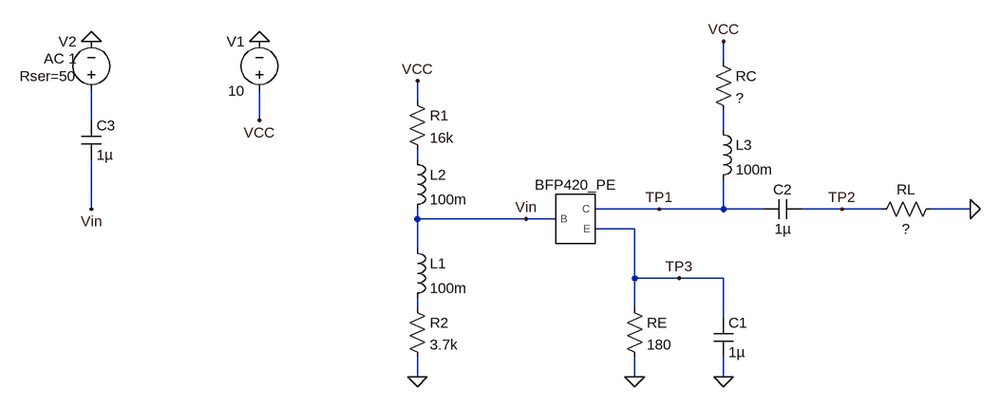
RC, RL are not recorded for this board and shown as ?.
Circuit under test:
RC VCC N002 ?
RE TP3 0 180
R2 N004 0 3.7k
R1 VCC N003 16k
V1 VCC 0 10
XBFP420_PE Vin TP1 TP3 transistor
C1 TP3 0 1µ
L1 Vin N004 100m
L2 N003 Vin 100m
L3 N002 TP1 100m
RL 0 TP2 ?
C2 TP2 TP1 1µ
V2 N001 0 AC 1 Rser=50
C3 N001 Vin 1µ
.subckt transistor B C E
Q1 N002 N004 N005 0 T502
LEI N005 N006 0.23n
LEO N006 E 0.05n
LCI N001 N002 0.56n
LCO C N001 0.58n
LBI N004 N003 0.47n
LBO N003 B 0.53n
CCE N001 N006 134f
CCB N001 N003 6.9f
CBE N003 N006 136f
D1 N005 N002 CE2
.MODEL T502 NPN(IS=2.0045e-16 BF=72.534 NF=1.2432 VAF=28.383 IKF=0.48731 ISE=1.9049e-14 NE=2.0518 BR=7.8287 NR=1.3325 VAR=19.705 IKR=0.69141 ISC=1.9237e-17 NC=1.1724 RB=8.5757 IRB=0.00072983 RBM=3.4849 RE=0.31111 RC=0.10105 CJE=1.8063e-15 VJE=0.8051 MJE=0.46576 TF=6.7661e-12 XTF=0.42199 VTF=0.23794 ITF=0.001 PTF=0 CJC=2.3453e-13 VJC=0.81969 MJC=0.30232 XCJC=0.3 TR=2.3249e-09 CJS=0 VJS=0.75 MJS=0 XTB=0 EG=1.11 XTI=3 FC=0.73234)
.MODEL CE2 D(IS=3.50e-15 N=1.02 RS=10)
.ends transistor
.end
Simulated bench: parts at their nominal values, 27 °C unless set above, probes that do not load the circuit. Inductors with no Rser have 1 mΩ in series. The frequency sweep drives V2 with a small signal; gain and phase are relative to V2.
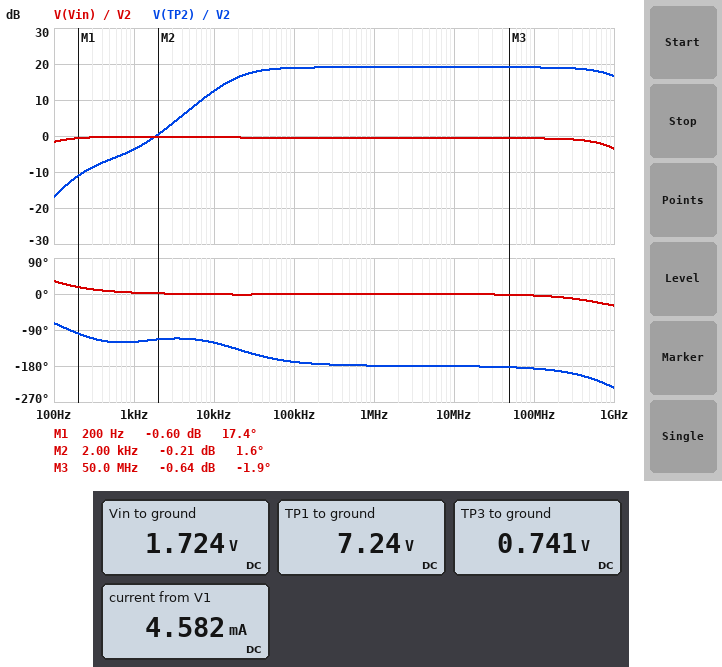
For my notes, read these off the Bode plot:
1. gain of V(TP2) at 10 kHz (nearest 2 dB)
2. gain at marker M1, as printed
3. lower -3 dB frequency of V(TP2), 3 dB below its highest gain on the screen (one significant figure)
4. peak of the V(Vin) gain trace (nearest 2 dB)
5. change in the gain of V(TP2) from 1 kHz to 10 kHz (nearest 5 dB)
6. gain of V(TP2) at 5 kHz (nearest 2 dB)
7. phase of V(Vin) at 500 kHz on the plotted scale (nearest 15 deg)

12 dB
-0.60 dB
20 kHz
0 dB
15 dB
8 dB
0 deg
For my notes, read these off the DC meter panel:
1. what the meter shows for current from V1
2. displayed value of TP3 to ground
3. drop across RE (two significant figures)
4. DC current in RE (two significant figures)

4.582 mA
0.741 V
740 mV
4.1 mA
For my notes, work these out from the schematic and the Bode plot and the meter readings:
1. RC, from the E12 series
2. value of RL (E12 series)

680 Ω
82 Ω
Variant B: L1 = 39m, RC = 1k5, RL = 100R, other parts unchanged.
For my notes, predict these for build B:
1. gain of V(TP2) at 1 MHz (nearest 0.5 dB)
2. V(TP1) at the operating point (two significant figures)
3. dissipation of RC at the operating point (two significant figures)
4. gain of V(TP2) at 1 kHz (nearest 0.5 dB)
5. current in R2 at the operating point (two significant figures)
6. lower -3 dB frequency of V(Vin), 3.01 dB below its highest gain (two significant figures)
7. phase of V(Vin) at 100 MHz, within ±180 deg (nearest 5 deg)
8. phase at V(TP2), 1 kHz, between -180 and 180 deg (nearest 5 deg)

20.5 dB
4.0 V
24 mW
-2.5 dB
460 µA
64 Hz
-5 deg
-125 deg
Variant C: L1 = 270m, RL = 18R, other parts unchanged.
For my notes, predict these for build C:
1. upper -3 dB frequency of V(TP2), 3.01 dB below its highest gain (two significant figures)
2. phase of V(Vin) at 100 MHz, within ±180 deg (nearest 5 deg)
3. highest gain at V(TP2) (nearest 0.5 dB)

2.3 GHz
0 deg
6.0 dB
